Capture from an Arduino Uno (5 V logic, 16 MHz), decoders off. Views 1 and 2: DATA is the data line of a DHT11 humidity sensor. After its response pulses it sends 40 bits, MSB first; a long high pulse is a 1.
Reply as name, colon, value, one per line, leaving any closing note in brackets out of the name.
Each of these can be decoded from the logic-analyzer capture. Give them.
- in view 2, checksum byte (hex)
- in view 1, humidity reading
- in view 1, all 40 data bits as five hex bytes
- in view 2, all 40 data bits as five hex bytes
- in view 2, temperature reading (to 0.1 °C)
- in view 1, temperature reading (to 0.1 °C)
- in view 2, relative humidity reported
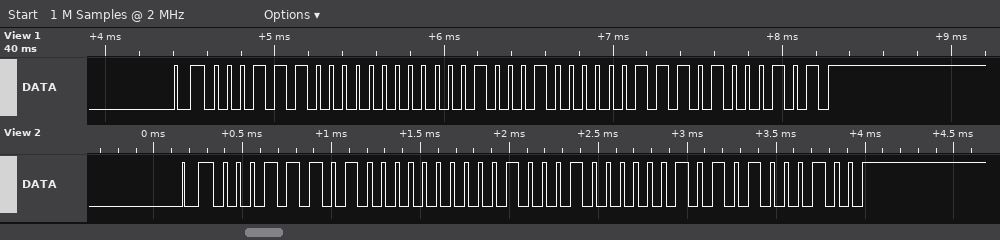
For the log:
in view 2, checksum byte: 0x44
in view 1, humidity reading: 28 %
in view 1, all 40 data bits as five hex bytes: 1C 00 22 07 45
in view 2, all 40 data bits as five hex bytes: 1D 00 22 05 44
in view 2, temperature reading: 34.5 °C
in view 1, temperature reading: 34.7 °C
in view 2, relative humidity reported: 29 %
